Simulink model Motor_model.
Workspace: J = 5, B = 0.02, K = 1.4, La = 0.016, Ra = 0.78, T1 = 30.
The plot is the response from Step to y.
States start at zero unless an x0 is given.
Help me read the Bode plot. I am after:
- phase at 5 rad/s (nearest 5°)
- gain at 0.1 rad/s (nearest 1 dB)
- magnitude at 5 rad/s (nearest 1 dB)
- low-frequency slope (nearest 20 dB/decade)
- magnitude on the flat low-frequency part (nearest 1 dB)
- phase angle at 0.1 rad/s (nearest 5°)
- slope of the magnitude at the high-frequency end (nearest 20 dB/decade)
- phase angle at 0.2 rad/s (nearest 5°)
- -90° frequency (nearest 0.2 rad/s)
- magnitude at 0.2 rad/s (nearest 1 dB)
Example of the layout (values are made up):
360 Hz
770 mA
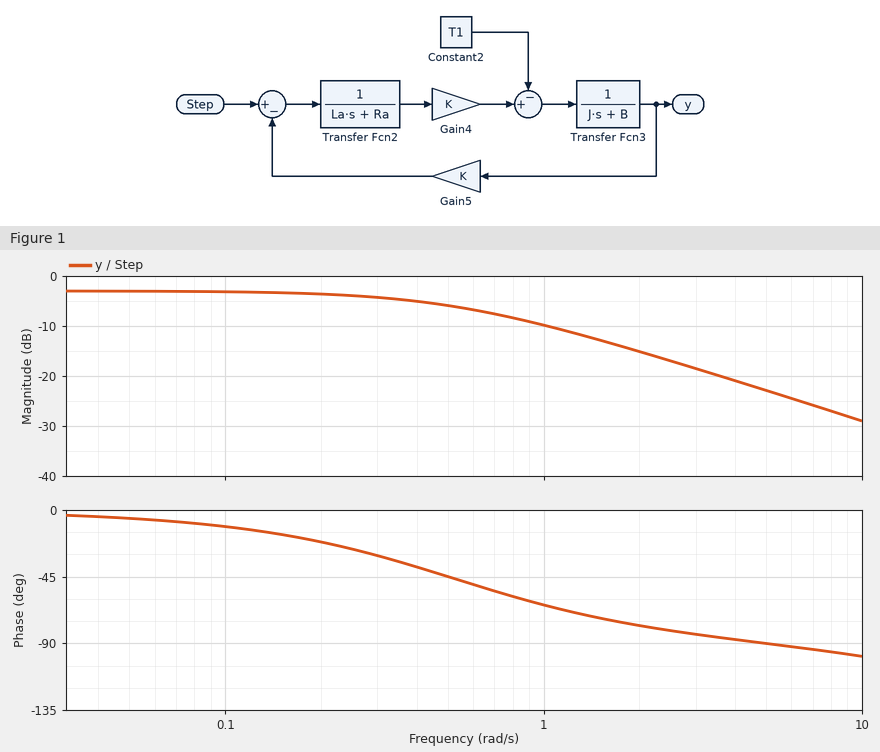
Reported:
-90°
-3 dB
-23 dB
0 dB/decade
-3 dB
-10°
-20 dB/decade
-20°
5.0 rad/s
-4 dB
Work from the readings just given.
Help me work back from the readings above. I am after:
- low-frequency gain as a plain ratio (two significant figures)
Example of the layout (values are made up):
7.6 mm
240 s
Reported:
0.71
